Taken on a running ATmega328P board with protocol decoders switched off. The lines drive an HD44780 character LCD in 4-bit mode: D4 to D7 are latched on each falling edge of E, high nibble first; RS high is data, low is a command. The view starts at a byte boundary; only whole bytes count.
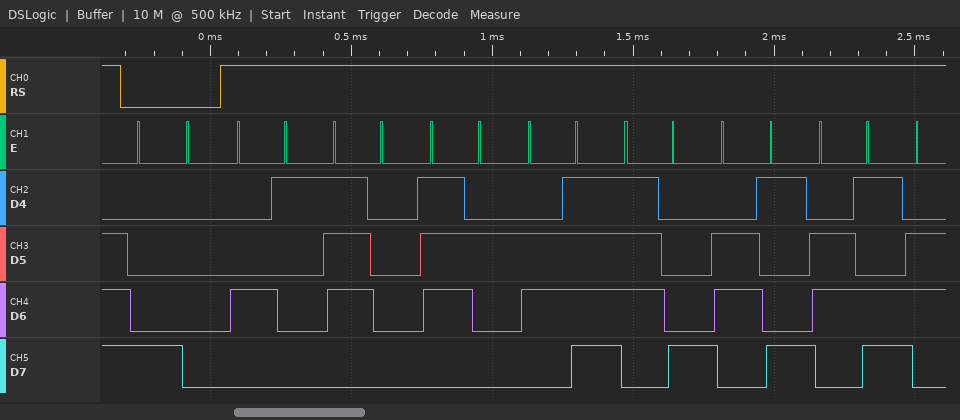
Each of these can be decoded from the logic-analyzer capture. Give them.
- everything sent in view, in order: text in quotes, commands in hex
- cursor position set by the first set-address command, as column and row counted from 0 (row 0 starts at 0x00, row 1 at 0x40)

0x80 "Aproxim"
column 0, row 0
